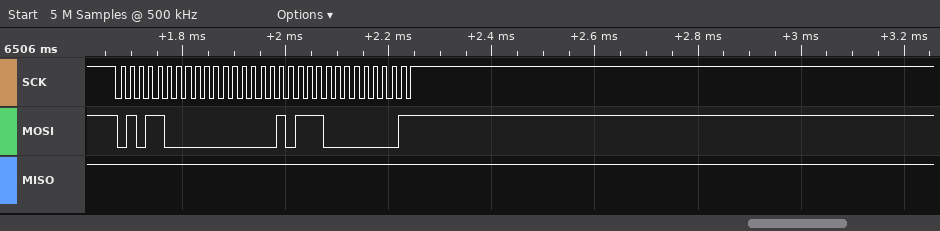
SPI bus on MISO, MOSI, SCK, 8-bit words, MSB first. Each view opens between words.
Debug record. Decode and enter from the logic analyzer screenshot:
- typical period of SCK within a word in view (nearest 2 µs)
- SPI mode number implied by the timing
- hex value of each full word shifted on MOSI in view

18 µs
3
58, 00, 5C, 03
